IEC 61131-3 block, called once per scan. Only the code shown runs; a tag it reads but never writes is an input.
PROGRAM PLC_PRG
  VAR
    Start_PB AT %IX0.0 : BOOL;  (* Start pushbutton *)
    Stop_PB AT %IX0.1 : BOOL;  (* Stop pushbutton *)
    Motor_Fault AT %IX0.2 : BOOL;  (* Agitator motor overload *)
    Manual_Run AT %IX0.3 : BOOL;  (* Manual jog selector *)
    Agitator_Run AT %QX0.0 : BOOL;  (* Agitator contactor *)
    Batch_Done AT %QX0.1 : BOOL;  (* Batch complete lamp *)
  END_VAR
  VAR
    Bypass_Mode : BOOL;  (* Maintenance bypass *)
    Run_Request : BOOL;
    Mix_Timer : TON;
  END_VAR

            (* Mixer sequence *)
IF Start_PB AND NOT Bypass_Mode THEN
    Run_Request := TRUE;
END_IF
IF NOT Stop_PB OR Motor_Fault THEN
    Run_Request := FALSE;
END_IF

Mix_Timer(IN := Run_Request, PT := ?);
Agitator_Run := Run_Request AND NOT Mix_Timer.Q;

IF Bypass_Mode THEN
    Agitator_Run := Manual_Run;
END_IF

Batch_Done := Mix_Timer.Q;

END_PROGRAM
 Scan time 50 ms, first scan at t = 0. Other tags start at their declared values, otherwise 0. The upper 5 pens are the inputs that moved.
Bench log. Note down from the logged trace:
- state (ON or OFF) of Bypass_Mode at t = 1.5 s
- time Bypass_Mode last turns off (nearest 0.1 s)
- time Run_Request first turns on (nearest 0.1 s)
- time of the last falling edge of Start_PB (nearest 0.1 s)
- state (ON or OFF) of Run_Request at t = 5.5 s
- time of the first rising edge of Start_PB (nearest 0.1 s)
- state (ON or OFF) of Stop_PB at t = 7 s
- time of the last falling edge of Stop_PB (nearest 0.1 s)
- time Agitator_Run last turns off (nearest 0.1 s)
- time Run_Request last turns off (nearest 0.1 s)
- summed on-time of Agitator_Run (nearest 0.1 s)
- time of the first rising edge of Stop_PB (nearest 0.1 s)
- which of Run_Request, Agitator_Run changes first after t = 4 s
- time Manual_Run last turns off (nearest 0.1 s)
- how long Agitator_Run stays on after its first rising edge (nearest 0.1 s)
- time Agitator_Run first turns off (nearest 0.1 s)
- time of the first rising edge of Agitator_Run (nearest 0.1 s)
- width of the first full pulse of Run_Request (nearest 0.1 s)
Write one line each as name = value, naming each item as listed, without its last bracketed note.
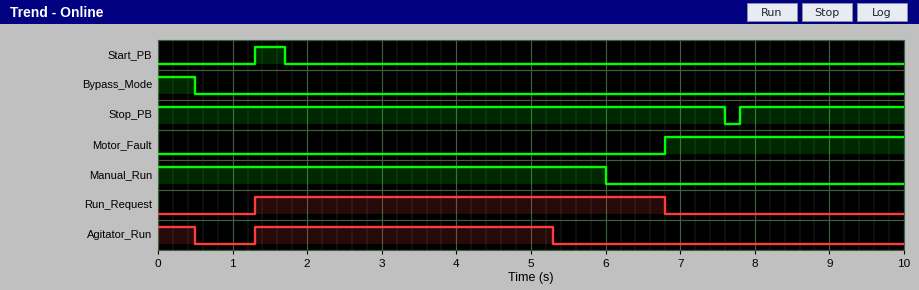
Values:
state (ON or OFF) of Bypass_Mode at t = 1.5 s = OFF
time Bypass_Mode last turns off = 0.5 s
time Run_Request first turns on = 1.3 s
time of the last falling edge of Start_PB = 1.7 s
state (ON or OFF) of Run_Request at t = 5.5 s = ON
time of the first rising edge of Start_PB = 1.3 s
state (ON or OFF) of Stop_PB at t = 7 s = ON
time of the last falling edge of Stop_PB = 7.6 s
time Agitator_Run last turns off = 5.3 s
time Run_Request last turns off = 6.8 s
summed on-time of Agitator_Run = 4.5 s
time of the first rising edge of Stop_PB = 7.8 s
which of Run_Request, Agitator_Run changes first after t = 4 s = Agitator_Run
time Manual_Run last turns off = 6.0 s
how long Agitator_Run stays on after its first rising edge = 4.0 s
time Agitator_Run first turns off = 0.5 s
time of the first rising edge of Agitator_Run = 1.3 s
width of the first full pulse of Run_Request = 5.5 s
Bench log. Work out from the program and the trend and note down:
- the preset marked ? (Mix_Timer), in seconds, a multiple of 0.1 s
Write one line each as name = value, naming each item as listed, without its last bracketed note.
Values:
the preset marked ? (Mix_Timer), in seconds, a multiple of 0.1 s = 4.0 s
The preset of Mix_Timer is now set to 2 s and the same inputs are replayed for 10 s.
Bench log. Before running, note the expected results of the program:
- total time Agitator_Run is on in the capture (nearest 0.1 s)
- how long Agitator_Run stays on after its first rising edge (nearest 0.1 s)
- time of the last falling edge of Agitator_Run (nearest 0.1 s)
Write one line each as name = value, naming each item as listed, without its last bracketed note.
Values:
total time Agitator_Run is on in the capture = 2.5 s
how long Agitator_Run stays on after its first rising edge = 2.0 s
time of the last falling edge of Agitator_Run = 3.3 s
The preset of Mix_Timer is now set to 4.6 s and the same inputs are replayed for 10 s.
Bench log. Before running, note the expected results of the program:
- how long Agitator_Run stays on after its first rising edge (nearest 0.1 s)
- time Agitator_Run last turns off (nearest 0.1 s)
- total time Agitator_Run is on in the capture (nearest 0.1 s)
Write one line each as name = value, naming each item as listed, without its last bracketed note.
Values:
how long Agitator_Run stays on after its first rising edge = 4.6 s
time Agitator_Run last turns off = 5.9 s
total time Agitator_Run is on in the capture = 5.1 s
